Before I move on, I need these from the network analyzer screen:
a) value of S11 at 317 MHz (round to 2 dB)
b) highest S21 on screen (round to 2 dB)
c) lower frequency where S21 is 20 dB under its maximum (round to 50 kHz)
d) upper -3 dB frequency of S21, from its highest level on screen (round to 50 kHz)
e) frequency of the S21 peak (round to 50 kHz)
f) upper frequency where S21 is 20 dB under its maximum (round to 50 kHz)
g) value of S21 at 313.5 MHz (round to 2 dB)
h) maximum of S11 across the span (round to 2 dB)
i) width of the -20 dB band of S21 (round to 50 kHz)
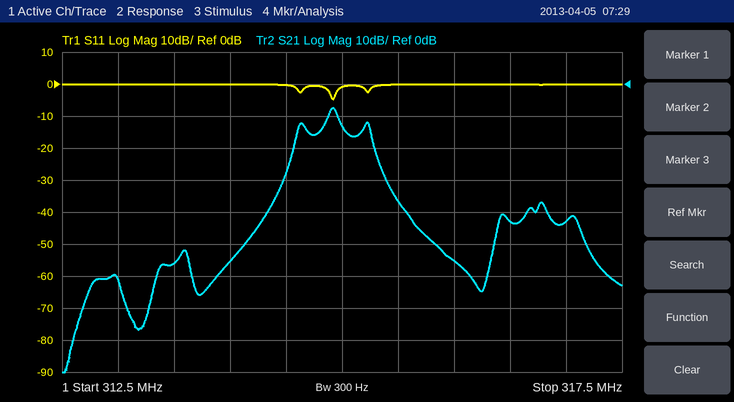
0 dB
-8 dB
314.50 MHz
314.95 MHz
314.90 MHz
315.35 MHz
-56 dB
0 dB
850 kHz
